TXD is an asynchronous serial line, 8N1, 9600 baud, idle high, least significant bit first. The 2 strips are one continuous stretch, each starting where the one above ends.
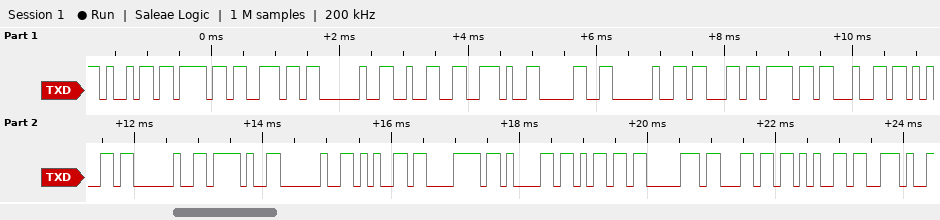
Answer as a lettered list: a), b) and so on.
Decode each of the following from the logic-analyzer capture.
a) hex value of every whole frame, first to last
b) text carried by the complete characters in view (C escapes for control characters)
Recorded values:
a) 69 6F 6E 20 32 2E 30 20 63 6F 64 65 20 2F 20 65 78 61 6D 70 6C 65 2E
b) "ion 2.0 code / example."
